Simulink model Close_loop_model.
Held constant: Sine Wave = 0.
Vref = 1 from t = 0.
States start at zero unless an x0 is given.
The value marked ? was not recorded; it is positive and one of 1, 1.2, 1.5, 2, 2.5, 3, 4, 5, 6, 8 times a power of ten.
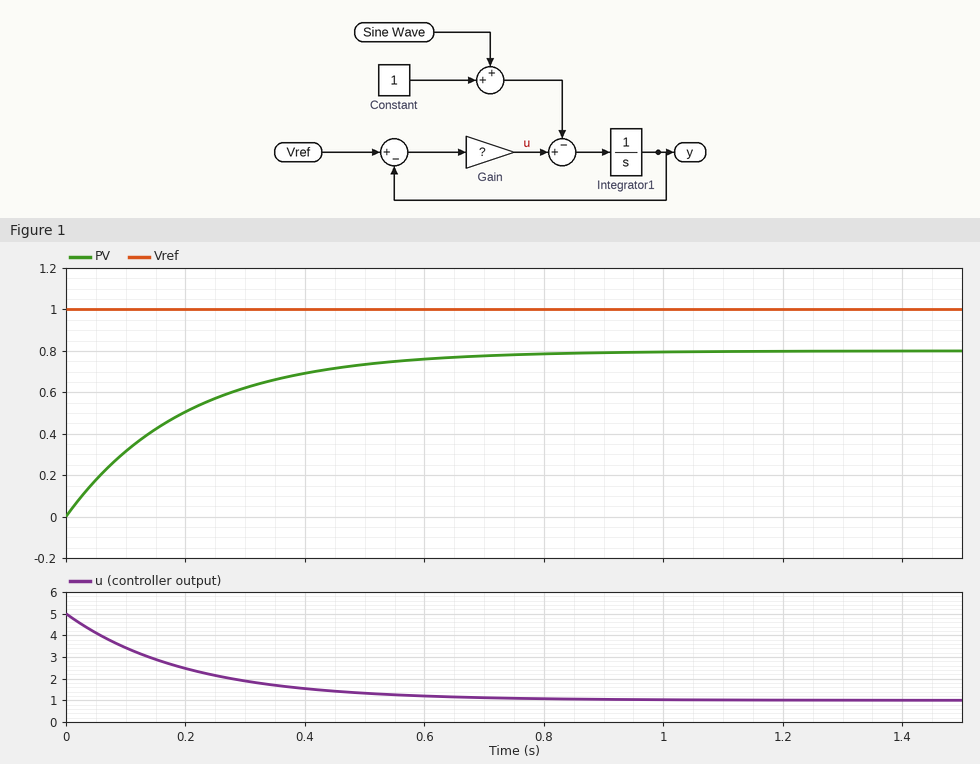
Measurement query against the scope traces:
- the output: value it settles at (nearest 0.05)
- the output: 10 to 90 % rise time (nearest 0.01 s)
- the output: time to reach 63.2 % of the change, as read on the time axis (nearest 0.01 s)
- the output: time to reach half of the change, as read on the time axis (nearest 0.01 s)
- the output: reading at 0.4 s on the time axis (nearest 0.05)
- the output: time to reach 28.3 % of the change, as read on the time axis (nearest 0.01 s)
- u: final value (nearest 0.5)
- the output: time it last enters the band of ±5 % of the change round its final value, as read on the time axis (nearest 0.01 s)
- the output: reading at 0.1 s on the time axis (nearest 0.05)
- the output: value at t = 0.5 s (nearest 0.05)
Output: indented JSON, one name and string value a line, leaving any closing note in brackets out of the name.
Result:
{
  "the output: value it settles at": "0.80",
  "the output: 10 to 90 % rise time": "0.44 s",
  "the output: time to reach 63.2 % of the change, as read on the time axis": "0.20 s",
  "the output: time to reach half of the change, as read on the time axis": "0.14 s",
  "the output: reading at 0.4 s on the time axis": "0.70",
  "the output: time to reach 28.3 % of the change, as read on the time axis": "0.07 s",
  "u: final value": "1.0",
  "the output: time it last enters the band of ±5 % of the change round its final value, as read on the time axis": "0.60 s",
  "the output: reading at 0.1 s on the time axis": "0.30",
  "the output: value at t = 0.5 s": "0.75"
}
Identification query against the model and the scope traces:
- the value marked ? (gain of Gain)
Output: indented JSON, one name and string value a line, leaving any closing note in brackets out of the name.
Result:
{
  "the value marked ?": "5"
}
